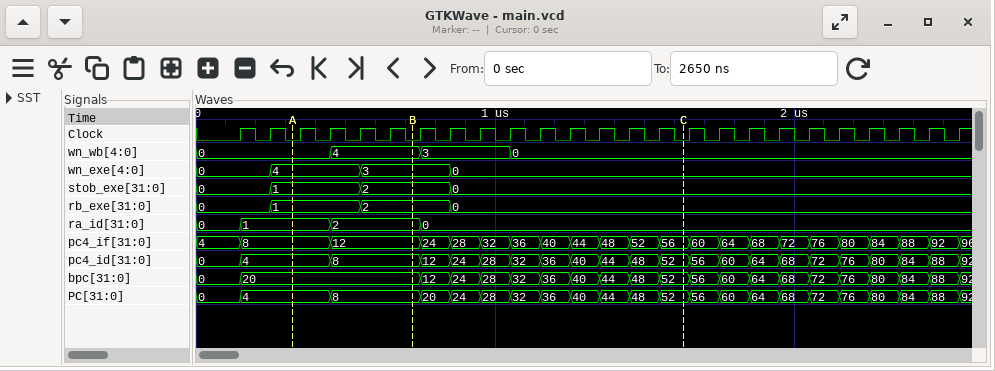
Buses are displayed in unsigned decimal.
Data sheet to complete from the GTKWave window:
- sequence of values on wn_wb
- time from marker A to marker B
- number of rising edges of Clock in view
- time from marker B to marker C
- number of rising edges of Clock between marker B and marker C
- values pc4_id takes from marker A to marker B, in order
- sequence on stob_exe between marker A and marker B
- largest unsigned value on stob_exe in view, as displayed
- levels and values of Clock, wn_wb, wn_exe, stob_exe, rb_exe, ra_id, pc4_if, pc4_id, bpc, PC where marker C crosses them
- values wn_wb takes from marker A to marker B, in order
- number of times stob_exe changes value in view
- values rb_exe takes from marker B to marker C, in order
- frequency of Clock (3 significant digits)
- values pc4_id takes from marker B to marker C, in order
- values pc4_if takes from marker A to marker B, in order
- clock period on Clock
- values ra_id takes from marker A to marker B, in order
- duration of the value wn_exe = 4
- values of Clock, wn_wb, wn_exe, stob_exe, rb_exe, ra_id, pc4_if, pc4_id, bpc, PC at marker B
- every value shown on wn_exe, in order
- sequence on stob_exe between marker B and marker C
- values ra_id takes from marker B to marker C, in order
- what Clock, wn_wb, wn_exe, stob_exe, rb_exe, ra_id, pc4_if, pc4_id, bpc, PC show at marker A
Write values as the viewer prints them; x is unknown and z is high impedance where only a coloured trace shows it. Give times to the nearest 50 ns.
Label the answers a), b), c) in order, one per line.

a) 0, 4, 3, 0
b) 400 ns
c) 25
d) 900 ns
e) 9
f) 4, 8
g) 1, 2
h) 2
i) Clock=0, wn_wb=0, wn_exe=0, stob_exe=0, rb_exe=0, ra_id=0, pc4_if=56, pc4_id=52, bpc=52, PC=52
j) 0, 4
k) 3
l) 2, 0
m) 10.0 MHz
n) 8, 12, 24, 28, 32, 36, 40, 44, 48, 52
o) 8, 12
p) 100 ns
q) 1, 2
r) 300 ns
s) Clock=0, wn_wb=4, wn_exe=3, stob_exe=2, rb_exe=2, ra_id=2, pc4_if=12, pc4_id=8, bpc=20, PC=8
t) 0, 4, 3, 0
u) 2, 0
v) 2, 0
w) Clock=0, wn_wb=0, wn_exe=4, stob_exe=1, rb_exe=1, ra_id=1, pc4_if=8, pc4_id=4, bpc=20, PC=4
